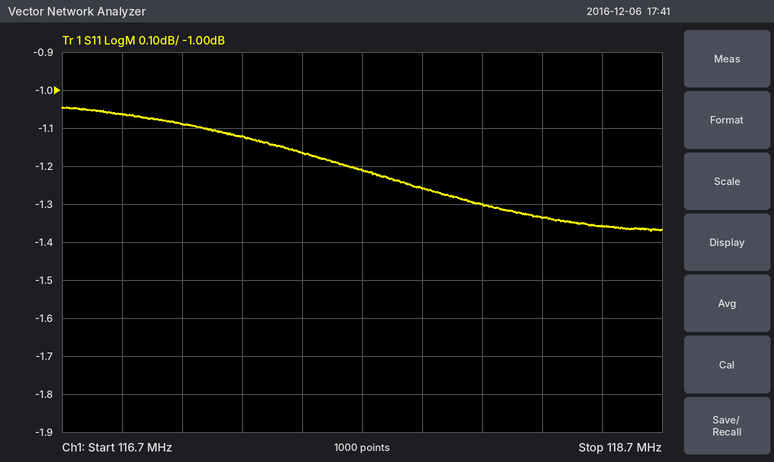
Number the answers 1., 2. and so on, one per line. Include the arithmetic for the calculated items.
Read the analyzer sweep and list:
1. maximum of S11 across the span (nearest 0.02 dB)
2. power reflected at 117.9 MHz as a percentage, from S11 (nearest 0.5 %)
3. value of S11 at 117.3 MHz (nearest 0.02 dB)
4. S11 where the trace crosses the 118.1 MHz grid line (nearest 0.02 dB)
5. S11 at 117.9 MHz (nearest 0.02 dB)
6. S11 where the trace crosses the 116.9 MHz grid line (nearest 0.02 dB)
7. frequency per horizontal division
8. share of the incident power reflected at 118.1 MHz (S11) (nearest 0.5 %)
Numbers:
1. -1.04 dB
2. 10^(-1.26/10) ≈ 74.8 %, so 75.0 % to the nearest 0.5 %
3. -1.12 dB
4. -1.30 dB
5. -1.26 dB
6. -1.06 dB
7. 200 kHz
8. 10^(-1.3/10) ≈ 74.1 %, so 74.0 % to the nearest 0.5 %
